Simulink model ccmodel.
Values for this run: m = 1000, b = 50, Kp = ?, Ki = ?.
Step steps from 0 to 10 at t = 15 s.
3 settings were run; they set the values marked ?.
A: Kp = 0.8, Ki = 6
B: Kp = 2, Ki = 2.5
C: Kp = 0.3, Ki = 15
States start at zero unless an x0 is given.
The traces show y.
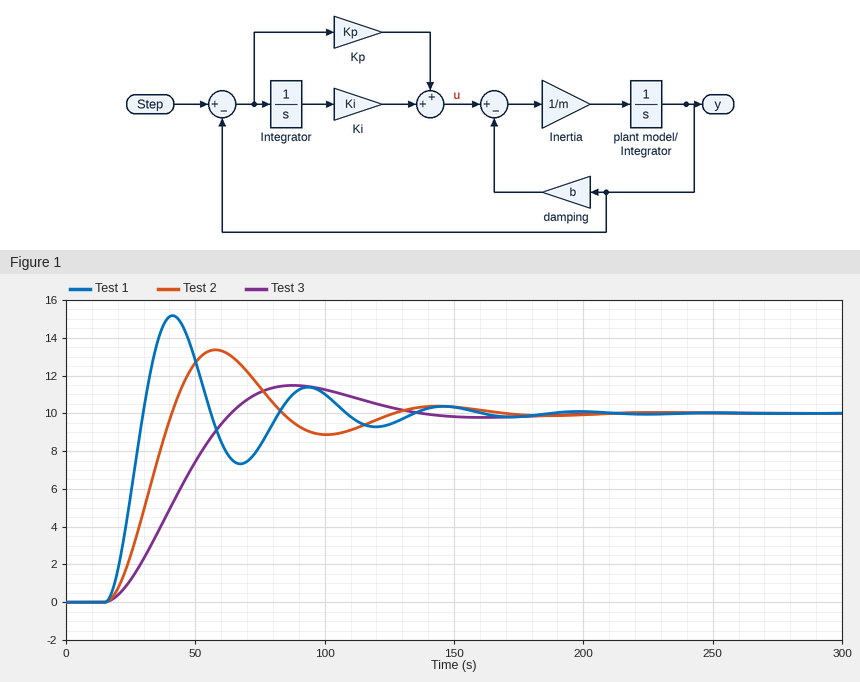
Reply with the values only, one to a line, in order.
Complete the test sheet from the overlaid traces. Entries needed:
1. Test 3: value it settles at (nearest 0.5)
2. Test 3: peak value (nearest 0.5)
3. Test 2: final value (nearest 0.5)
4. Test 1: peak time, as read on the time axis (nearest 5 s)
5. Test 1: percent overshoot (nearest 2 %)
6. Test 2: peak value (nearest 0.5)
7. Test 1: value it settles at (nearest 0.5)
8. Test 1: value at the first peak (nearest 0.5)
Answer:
10.0
11.5
10.0
40 s
52 %
13.5
10.0
15.0
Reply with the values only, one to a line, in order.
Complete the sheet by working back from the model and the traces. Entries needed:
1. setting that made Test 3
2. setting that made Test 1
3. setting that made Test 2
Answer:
B
C
A
